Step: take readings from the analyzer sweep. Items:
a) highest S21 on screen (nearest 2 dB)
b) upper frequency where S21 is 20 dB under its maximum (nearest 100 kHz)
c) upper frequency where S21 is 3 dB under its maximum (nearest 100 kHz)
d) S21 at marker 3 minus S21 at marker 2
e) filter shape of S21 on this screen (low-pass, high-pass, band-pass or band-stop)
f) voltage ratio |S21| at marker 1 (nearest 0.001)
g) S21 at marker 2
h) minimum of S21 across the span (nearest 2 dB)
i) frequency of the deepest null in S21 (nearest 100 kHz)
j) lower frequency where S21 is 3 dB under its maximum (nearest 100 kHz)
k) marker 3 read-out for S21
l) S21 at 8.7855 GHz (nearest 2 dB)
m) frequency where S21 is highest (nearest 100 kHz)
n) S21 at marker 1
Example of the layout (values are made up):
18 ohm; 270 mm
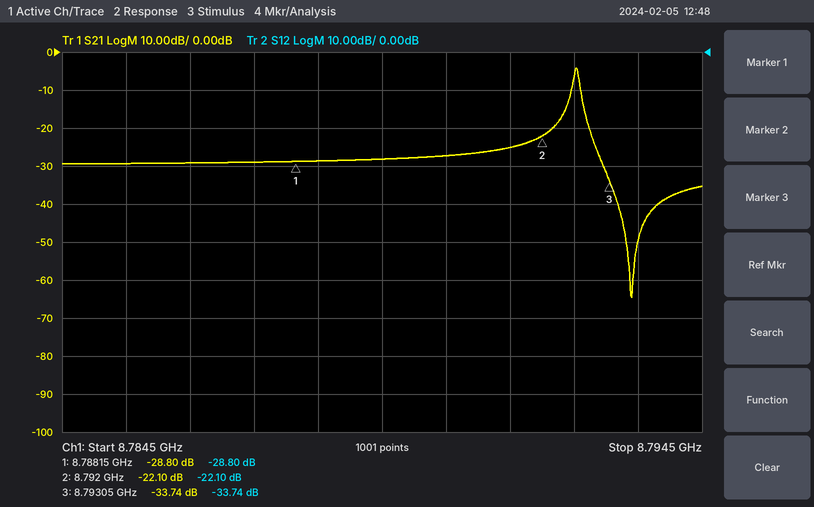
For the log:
-4 dB; 8.7928 GHz; 8.7926 GHz; -11.64 dB; band-pass; 0.036; -22.10 dB; -64 dB; 8.7934 GHz; 8.7925 GHz; -33.74 dB; -30 dB; 8.7925 GHz; -28.80 dB
